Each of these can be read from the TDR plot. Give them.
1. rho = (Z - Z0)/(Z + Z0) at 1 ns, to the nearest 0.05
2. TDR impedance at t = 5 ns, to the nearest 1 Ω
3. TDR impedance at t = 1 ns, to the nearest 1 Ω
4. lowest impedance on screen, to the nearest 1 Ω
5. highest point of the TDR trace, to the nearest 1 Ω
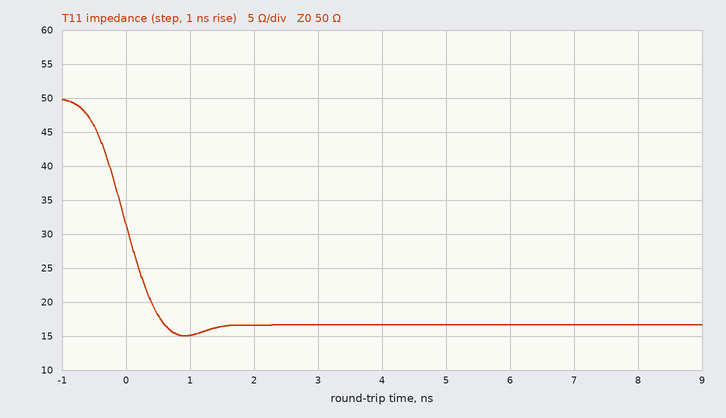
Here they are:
-0.55
17 Ω
15 Ω
15 Ω
50 Ω
